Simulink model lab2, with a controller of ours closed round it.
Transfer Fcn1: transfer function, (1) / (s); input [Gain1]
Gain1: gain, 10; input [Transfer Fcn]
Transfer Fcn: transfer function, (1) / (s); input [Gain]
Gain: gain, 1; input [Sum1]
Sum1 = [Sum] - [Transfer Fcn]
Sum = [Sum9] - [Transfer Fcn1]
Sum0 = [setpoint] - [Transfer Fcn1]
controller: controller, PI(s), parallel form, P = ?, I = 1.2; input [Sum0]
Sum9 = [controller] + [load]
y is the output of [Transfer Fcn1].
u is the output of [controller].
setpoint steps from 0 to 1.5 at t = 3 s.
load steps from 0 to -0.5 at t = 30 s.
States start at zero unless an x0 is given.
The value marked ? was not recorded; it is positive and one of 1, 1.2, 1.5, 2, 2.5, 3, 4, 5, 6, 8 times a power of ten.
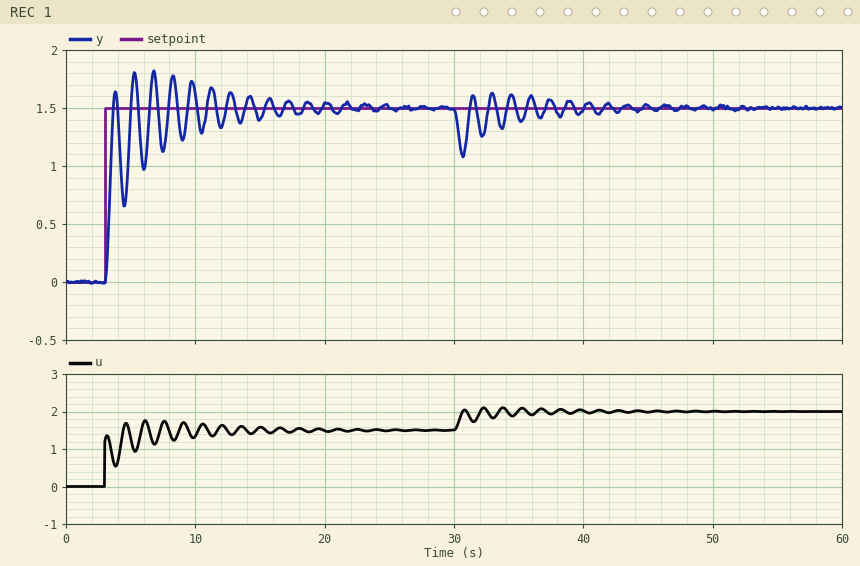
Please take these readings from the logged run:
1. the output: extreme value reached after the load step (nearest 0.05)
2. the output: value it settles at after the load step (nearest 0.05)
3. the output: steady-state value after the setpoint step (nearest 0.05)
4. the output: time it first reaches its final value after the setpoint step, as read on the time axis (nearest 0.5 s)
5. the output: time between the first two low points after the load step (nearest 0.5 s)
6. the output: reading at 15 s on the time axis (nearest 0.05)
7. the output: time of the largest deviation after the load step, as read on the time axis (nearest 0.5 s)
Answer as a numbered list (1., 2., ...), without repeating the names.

1. 1.10
2. 1.50
3. 1.50
4. 3.5 s
5. 1.5 s
6. 1.40
7. 30.5 s
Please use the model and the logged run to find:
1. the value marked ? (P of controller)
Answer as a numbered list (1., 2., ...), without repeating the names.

1. 0.8
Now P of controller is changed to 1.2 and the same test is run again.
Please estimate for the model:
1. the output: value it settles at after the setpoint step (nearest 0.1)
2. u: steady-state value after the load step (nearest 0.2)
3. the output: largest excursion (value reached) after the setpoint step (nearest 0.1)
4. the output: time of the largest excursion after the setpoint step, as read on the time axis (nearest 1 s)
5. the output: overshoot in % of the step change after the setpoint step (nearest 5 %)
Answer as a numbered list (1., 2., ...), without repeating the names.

1. 1.5
2. 2.0
3. 1.8
4. 5 s
5. 20 %
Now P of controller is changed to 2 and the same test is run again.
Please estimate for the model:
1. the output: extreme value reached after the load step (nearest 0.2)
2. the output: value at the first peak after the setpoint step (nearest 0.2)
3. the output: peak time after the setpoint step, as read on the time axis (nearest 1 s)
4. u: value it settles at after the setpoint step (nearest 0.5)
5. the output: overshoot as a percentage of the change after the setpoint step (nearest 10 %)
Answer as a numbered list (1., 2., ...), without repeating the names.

1. 1.2
2. 2.0
3. 4 s
4. 1.5
5. 30 %
